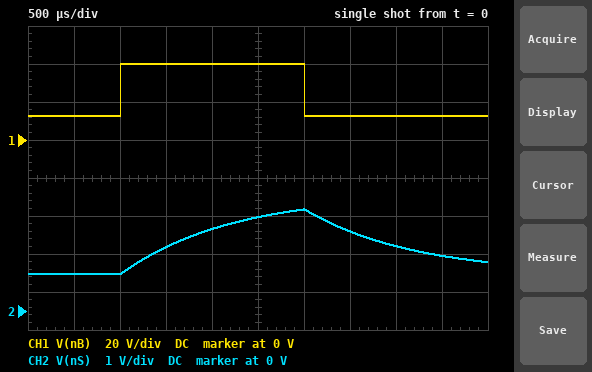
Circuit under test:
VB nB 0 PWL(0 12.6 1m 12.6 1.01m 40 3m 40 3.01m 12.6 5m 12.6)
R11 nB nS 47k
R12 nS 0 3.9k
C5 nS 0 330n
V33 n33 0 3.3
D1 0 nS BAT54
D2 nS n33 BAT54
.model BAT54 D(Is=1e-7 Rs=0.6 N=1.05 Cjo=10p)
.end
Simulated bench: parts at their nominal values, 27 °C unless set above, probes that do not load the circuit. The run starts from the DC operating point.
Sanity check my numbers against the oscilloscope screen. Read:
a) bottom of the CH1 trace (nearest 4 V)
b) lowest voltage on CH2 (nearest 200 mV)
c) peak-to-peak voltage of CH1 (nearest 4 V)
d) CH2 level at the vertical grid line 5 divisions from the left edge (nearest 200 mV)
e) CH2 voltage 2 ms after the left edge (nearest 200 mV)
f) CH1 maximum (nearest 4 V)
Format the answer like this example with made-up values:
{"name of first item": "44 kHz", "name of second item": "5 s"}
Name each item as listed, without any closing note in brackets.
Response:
{"bottom of the CH1 trace": "12 V", "lowest voltage on CH2": "1.0 V", "peak-to-peak voltage of CH1": "28 V", "CH2 level at the vertical grid line 5 divisions from the left edge": "2.4 V", "CH2 voltage 2 ms after the left edge": "2.2 V", "CH1 maximum": "40 V"}
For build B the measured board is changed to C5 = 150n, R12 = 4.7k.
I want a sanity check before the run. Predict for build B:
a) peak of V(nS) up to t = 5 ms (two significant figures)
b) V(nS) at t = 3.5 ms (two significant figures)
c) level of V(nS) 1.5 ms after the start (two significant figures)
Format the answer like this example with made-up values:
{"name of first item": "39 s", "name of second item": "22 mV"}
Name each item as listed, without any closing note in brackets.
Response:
{"peak of V(nS) up to t = 5 ms": "3.5 V", "V(nS) at t = 3.5 ms": "2.2 V", "level of V(nS) 1.5 ms after the start": "2.5 V"}
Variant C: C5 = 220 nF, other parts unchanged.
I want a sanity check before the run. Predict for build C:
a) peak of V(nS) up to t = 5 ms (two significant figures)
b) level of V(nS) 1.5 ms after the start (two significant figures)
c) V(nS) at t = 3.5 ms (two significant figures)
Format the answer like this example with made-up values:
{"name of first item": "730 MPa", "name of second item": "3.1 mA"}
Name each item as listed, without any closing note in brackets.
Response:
{"peak of V(nS) up to t = 5 ms": "2.9 V", "level of V(nS) 1.5 ms after the start": "1.9 V", "V(nS) at t = 3.5 ms": "2.0 V"}
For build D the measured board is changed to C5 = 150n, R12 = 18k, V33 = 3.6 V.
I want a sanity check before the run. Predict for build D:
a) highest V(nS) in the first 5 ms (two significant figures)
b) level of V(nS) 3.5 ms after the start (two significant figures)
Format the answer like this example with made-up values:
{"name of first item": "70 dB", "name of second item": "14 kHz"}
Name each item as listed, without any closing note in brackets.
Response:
{"highest V(nS) in the first 5 ms": "3.8 V", "level of V(nS) 3.5 ms after the start": "3.7 V"}
